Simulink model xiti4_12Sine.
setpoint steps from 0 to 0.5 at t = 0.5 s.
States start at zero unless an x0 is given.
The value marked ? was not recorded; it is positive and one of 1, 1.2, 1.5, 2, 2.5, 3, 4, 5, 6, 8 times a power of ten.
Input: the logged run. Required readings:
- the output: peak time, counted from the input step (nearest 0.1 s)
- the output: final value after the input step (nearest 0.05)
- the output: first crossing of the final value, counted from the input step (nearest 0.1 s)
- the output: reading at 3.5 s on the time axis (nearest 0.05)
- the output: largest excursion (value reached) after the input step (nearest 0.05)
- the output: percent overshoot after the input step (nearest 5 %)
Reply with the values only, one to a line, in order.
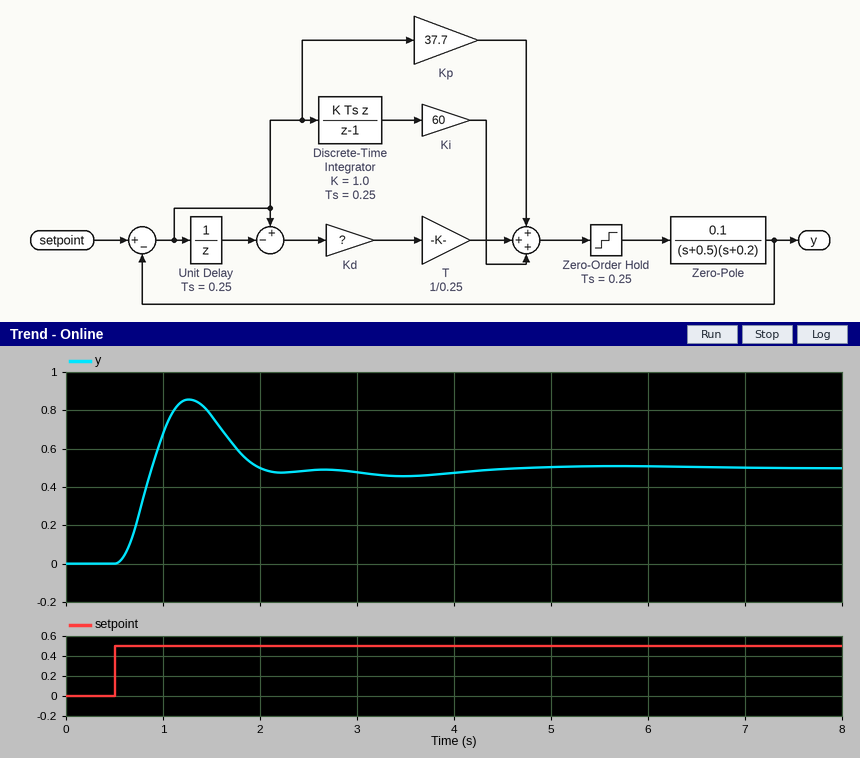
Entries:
0.8 s
0.50
0.4 s
0.45
0.85
70 %
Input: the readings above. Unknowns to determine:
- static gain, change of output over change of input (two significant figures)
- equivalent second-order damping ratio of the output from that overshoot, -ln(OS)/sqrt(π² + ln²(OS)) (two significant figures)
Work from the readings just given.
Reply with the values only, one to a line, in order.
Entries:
1.0
0.11
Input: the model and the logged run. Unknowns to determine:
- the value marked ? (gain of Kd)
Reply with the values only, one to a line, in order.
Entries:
30
